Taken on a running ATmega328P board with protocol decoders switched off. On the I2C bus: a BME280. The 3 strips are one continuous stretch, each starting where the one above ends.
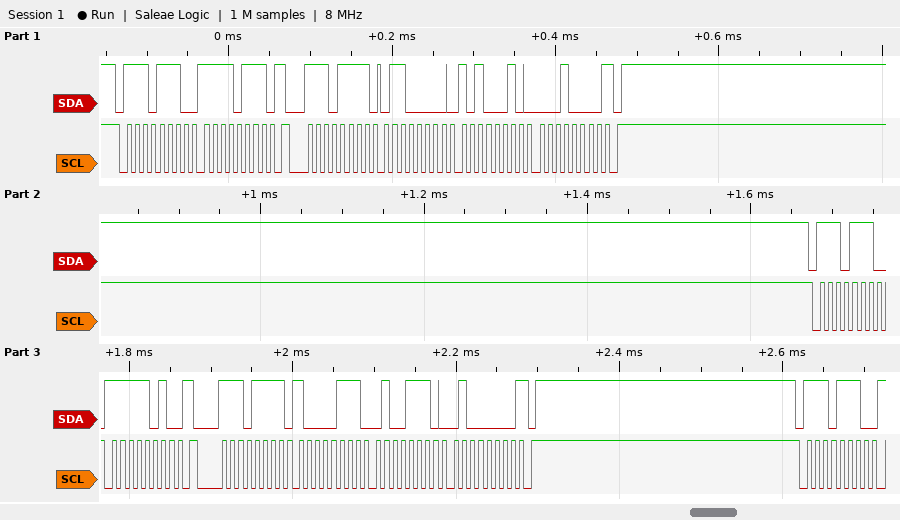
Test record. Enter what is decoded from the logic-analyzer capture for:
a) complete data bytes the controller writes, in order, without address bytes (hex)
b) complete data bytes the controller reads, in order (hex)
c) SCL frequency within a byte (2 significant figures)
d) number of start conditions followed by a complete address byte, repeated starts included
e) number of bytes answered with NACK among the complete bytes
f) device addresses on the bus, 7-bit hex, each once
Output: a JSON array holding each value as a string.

["F7 FA", "60 A2 10 87 4E 40", "100 kHz", "5", "2", "0x77"]
